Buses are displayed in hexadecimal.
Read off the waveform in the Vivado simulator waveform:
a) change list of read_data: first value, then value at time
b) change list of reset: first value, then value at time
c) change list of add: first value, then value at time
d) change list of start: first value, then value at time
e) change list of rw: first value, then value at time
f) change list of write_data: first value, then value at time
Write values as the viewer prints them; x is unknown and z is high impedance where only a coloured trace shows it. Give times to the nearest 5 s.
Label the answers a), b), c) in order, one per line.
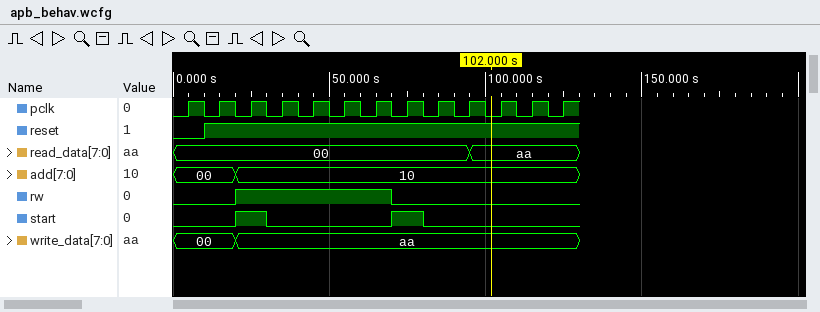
a) 00, aa at 95 s
b) 0, 1 at 10 s
c) 00, 10 at 20 s
d) 0, 1 at 20 s, 0 at 30 s, 1 at 70 s, 0 at 80 s
e) 0, 1 at 20 s, 0 at 70 s
f) 00, aa at 20 s
